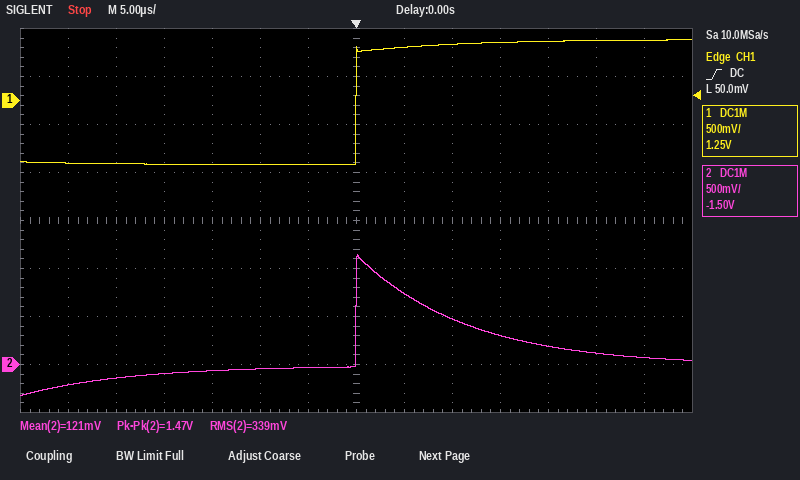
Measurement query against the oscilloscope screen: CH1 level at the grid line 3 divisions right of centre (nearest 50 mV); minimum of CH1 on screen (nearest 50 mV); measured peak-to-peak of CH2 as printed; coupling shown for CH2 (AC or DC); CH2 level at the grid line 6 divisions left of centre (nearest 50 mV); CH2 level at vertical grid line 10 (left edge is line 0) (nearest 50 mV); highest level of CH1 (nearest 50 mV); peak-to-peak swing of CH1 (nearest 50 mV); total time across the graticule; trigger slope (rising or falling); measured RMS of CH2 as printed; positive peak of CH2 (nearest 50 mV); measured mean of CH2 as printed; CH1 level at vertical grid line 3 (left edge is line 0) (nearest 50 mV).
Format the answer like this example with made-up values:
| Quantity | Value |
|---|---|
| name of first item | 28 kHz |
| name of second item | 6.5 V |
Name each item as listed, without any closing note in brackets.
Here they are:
| Quantity | Value |
|---|---|
| CH1 level at the grid line 3 divisions right of centre | 600 mV |
| minimum of CH1 on screen | -650 mV |
| measured peak-to-peak of CH2 as printed | 1.47 V |
| coupling shown for CH2 | DC |
| CH2 level at the grid line 6 divisions left of centre | -200 mV |
| CH2 level at vertical grid line 10 (left edge is line 0) | 300 mV |
| highest level of CH1 | 650 mV |
| peak-to-peak swing of CH1 | 1.30 V |
| total time across the graticule | 70 µs |
| trigger slope | rising |
| measured RMS of CH2 as printed | 339 mV |
| positive peak of CH2 | 1.15 V |
| measured mean of CH2 as printed | 121 mV |
| CH1 level at vertical grid line 3 (left edge is line 0) | -650 mV |
